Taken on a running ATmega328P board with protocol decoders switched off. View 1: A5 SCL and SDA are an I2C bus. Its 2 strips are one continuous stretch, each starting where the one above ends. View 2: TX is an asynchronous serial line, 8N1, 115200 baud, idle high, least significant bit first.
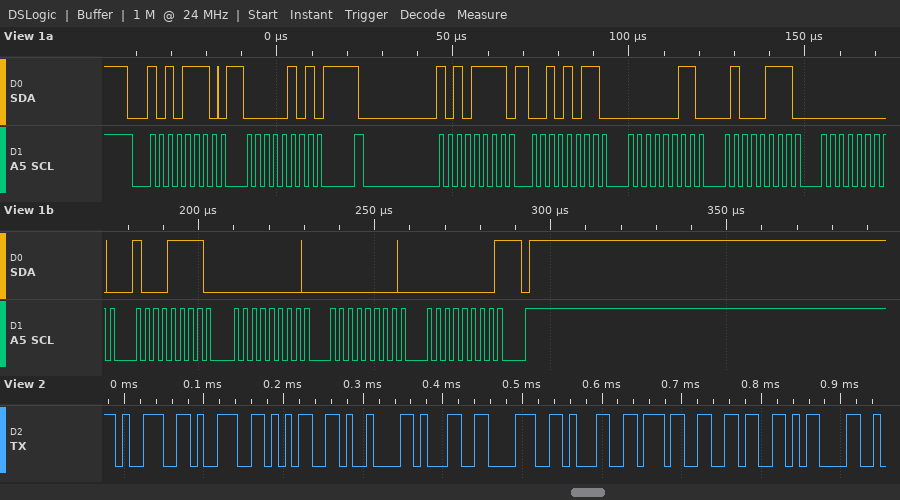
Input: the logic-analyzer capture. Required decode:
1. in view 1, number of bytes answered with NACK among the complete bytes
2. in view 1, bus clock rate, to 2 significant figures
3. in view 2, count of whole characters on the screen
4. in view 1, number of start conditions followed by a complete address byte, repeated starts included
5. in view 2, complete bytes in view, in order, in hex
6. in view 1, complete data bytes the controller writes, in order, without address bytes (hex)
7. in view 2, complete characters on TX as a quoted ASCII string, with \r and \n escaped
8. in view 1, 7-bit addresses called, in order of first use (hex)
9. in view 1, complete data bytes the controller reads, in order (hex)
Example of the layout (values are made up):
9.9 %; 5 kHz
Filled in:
1; 400 kHz; 10; 2; 39 39 35 09 31 38 31 37 36 0D; 05; "995\t18176\r"; 0x57; 2B 03 47 00 8F 00 00 00
